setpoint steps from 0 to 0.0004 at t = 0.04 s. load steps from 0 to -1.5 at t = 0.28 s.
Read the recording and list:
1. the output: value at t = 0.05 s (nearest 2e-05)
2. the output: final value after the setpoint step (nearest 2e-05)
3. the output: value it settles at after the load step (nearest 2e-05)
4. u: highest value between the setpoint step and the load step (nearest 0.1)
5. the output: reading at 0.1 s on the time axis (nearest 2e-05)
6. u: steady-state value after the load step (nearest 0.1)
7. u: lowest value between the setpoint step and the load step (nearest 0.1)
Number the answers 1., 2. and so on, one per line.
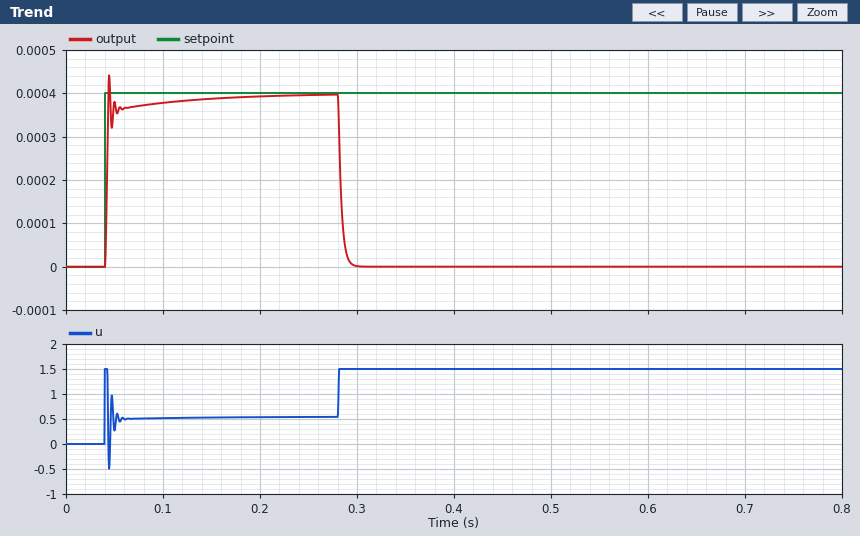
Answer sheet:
1. 0.00038
2. 0.00040
3. 0.00000
4. 1.5
5. 0.00038
6. 1.5
7. -0.5
